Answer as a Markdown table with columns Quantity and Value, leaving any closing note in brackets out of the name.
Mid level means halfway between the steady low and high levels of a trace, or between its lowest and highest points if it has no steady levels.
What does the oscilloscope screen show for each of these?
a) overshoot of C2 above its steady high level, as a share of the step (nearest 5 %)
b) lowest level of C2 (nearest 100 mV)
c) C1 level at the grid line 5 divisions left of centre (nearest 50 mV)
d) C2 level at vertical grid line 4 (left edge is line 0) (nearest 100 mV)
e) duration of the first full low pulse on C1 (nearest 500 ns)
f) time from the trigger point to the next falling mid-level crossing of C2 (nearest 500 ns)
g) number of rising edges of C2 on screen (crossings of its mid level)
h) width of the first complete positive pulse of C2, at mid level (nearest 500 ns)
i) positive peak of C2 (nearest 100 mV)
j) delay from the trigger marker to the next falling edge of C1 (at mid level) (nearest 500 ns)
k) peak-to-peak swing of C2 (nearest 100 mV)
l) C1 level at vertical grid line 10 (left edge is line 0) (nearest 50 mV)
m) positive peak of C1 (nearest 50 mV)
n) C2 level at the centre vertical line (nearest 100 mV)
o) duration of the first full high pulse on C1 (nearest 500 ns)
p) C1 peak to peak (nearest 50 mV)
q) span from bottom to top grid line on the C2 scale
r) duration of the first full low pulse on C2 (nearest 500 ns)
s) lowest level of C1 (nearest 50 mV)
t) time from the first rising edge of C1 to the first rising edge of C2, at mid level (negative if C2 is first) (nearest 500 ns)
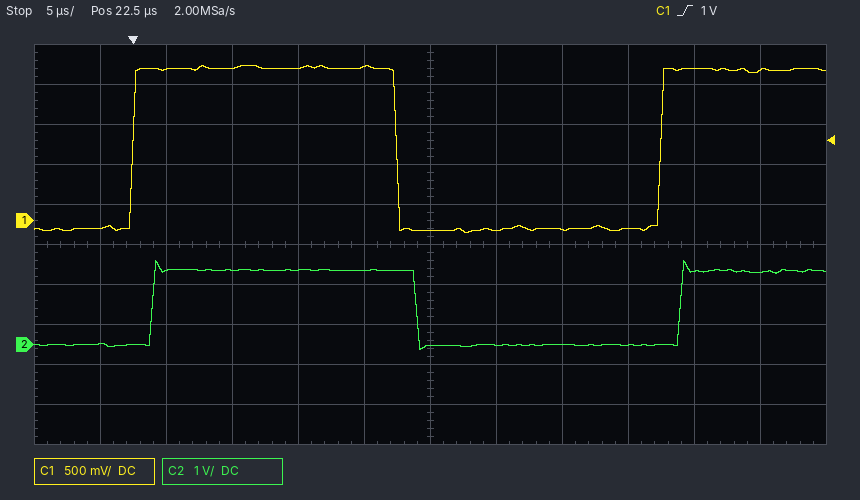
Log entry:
| Quantity | Value |
|---|---|
| overshoot of C2 above its steady high level, as a share of the step | 15 % |
| lowest level of C2 | -100 mV |
| C1 level at the grid line 5 divisions left of centre | -100 mV |
| C2 level at vertical grid line 4 (left edge is line 0) | 1.9 V |
| duration of the first full low pulse on C1 | 20.0 µs |
| time from the trigger point to the next falling mid-level crossing of C2 | 21.5 µs |
| number of rising edges of C2 on screen | 2 |
| width of the first complete positive pulse of C2, at mid level | 20.0 µs |
| positive peak of C2 | 2.1 V |
| delay from the trigger marker to the next falling edge of C1 (at mid level) | 20.0 µs |
| peak-to-peak swing of C2 | 2.2 V |
| C1 level at vertical grid line 10 (left edge is line 0) | 1.90 V |
| positive peak of C1 | 1.95 V |
| C2 level at the centre vertical line | 0.0 V |
| duration of the first full high pulse on C1 | 20.0 µs |
| C1 peak to peak | 2.10 V |
| span from bottom to top grid line on the C2 scale | 10 V |
| duration of the first full low pulse on C2 | 20.0 µs |
| lowest level of C1 | -150 mV |
| time from the first rising edge of C1 to the first rising edge of C2, at mid level (negative if C2 is first) | +1.5 µs |
